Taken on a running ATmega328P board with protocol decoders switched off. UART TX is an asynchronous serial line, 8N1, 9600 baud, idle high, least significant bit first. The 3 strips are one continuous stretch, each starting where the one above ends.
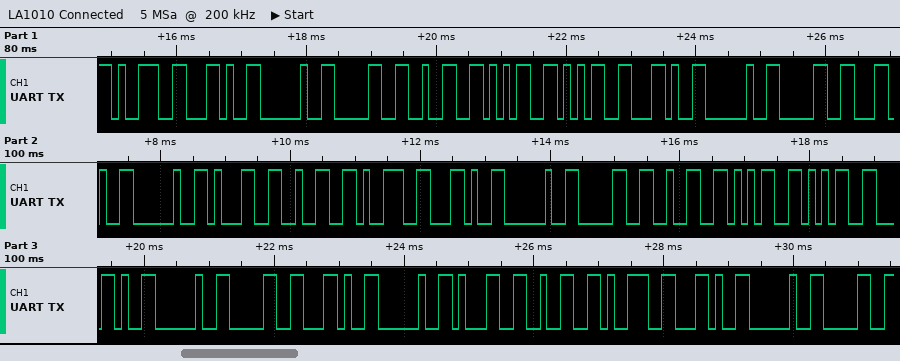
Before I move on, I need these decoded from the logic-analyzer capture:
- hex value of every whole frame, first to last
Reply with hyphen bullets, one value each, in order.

- 39 2C 20 30 32 35 35 2C 20 30 2C 20 31 32 39 2C 20 30 32 35 35 2C 20 30 2C 20 31 32 39 2C 20 30
